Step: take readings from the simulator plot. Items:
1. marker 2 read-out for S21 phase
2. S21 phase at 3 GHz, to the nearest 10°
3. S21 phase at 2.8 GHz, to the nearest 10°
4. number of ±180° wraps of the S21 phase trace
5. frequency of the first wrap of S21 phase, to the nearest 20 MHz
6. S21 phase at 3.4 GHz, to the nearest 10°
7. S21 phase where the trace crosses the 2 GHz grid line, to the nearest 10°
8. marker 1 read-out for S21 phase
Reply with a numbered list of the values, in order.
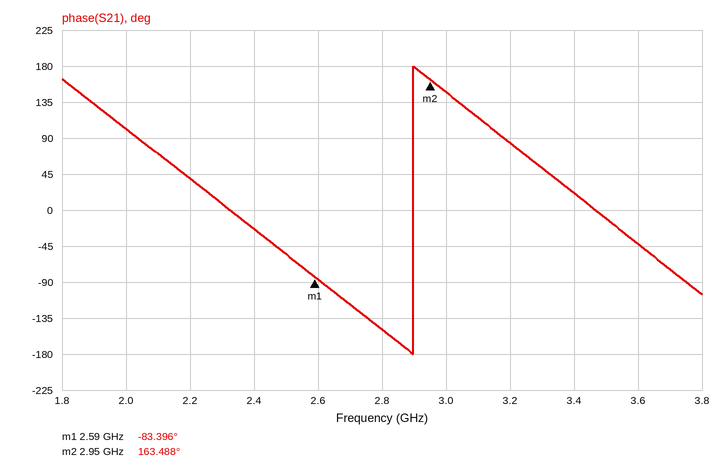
1. 163.488°
2. 150°
3. -150°
4. 1
5. 2.90 GHz
6. 20°
7. 100°
8. -83.396°
